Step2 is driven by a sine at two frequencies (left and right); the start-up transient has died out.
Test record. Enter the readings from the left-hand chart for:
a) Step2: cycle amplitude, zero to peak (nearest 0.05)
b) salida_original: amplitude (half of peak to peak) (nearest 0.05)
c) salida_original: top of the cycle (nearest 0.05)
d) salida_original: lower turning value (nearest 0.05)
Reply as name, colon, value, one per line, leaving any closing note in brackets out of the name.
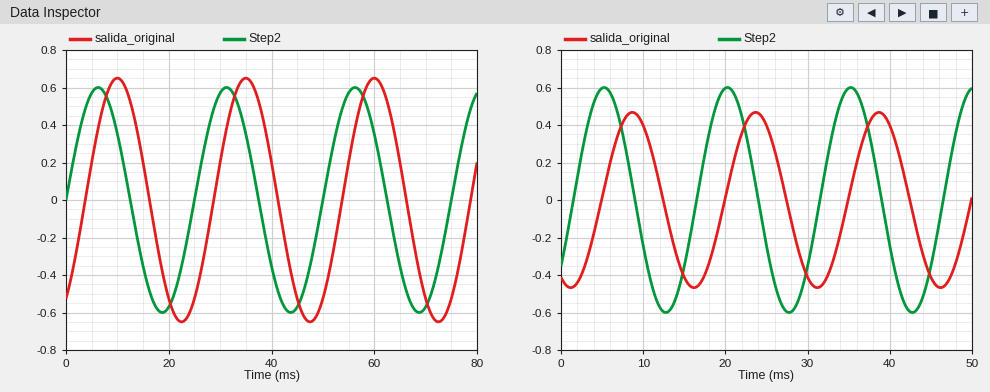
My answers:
Step2: cycle amplitude, zero to peak: 0.60
salida_original: amplitude (half of peak to peak): 0.65
salida_original: top of the cycle: 0.65
salida_original: lower turning value: -0.65
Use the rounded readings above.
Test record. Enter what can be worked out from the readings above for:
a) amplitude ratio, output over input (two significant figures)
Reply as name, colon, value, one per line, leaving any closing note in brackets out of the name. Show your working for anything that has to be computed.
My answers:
amplitude ratio, output over input: 0.65 / 0.6 = 1.1
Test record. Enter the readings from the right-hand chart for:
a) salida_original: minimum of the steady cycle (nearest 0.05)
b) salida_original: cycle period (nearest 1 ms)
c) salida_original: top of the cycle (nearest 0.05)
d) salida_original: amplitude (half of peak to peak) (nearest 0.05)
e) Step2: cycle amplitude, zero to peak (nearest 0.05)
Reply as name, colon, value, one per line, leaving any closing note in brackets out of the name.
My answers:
salida_original: minimum of the steady cycle: -0.45
salida_original: cycle period: 15 ms
salida_original: top of the cycle: 0.45
salida_original: amplitude (half of peak to peak): 0.45
Step2: cycle amplitude, zero to peak: 0.60
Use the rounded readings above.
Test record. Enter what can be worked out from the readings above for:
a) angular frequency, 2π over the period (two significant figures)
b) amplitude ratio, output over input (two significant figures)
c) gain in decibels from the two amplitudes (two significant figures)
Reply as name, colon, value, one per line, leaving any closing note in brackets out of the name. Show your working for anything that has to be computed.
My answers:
angular frequency, 2π over the period: 2π / 15 = 0.42 rad/ms
amplitude ratio, output over input: 0.45 / 0.6 = 0.75
gain in decibels from the two amplitudes: 20 log10(0.45 / 0.6) = -2.5 dB
